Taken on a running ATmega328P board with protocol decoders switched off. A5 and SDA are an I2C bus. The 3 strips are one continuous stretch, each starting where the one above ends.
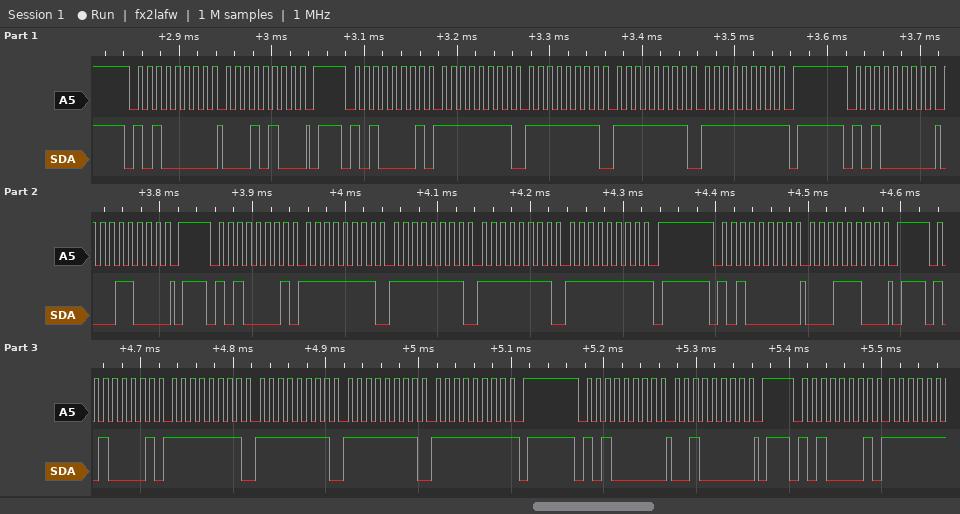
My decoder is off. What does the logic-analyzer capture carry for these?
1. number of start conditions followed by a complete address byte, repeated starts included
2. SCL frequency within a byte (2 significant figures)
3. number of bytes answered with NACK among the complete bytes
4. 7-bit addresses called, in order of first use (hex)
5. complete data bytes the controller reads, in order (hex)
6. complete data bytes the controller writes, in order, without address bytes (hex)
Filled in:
8
100 kHz
3
0x50
FF FF FF FF FF FF FF FF FF FF FF FF
14 18 1C 20
